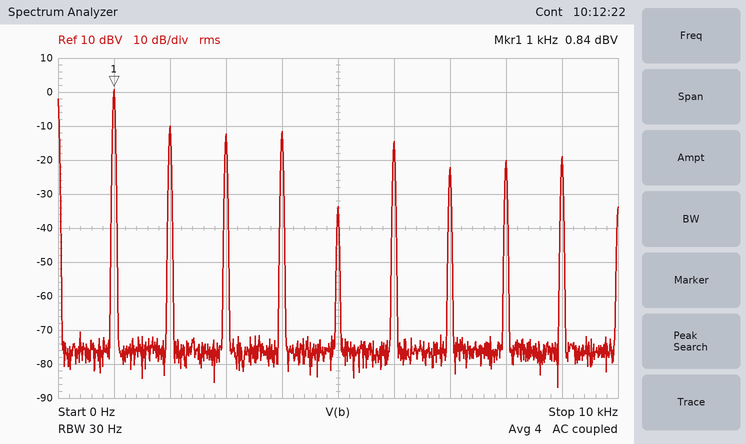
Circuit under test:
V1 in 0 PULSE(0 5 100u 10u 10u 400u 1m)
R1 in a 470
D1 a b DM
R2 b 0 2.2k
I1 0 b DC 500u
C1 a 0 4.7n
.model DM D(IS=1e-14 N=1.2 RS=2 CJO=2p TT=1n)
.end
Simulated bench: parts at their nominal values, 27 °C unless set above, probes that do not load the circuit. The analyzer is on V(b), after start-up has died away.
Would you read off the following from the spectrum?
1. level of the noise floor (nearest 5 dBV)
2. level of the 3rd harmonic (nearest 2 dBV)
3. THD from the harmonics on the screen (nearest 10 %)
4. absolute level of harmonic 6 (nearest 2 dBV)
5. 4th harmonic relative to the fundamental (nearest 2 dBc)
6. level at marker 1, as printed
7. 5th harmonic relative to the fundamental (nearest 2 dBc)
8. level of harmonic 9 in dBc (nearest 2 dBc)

-75 dBV
-12 dBV
50 %
-14 dBV
-12 dBc
0.84 dBV
-34 dBc
-20 dBc
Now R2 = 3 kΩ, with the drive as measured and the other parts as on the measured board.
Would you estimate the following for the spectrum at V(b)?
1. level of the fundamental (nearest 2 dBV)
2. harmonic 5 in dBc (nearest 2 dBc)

0 dBV
-36 dBc
